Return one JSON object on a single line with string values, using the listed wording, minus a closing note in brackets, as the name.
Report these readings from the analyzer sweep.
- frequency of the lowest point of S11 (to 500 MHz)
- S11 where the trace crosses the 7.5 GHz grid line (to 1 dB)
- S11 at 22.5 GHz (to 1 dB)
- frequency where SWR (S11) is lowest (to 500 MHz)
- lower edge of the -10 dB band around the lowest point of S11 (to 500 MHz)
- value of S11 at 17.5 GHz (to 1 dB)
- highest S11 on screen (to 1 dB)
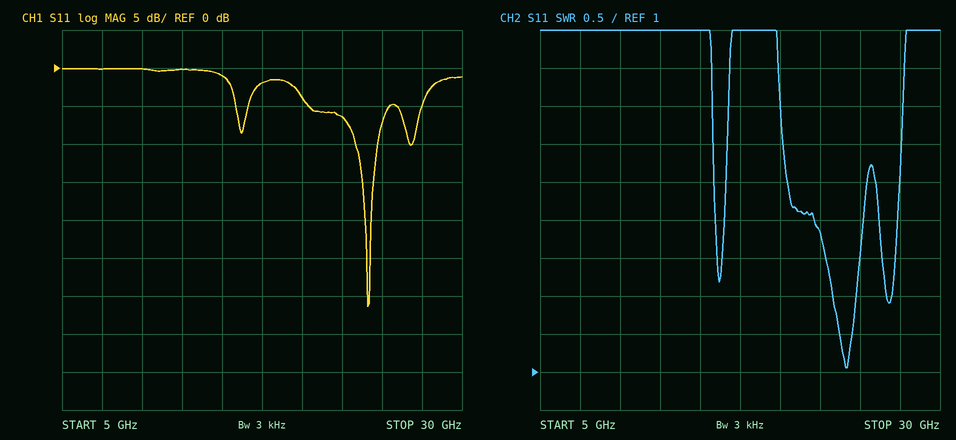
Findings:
{"frequency of the lowest point of S11": "24.0 GHz", "S11 where the trace crosses the 7.5 GHz grid line": "0 dB", "S11 at 22.5 GHz": "-6 dB", "frequency where SWR (S11) is lowest": "24.0 GHz", "lower edge of the -10 dB band around the lowest point of S11": "23.5 GHz", "value of S11 at 17.5 GHz": "-2 dB", "highest S11 on screen": "0 dB"}
